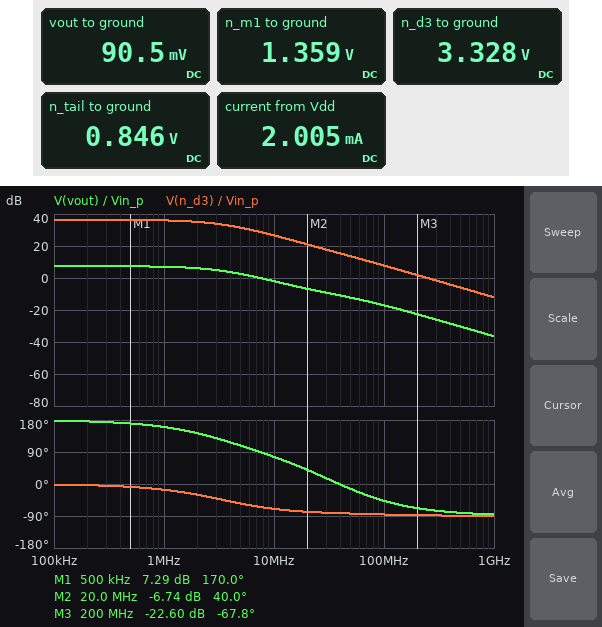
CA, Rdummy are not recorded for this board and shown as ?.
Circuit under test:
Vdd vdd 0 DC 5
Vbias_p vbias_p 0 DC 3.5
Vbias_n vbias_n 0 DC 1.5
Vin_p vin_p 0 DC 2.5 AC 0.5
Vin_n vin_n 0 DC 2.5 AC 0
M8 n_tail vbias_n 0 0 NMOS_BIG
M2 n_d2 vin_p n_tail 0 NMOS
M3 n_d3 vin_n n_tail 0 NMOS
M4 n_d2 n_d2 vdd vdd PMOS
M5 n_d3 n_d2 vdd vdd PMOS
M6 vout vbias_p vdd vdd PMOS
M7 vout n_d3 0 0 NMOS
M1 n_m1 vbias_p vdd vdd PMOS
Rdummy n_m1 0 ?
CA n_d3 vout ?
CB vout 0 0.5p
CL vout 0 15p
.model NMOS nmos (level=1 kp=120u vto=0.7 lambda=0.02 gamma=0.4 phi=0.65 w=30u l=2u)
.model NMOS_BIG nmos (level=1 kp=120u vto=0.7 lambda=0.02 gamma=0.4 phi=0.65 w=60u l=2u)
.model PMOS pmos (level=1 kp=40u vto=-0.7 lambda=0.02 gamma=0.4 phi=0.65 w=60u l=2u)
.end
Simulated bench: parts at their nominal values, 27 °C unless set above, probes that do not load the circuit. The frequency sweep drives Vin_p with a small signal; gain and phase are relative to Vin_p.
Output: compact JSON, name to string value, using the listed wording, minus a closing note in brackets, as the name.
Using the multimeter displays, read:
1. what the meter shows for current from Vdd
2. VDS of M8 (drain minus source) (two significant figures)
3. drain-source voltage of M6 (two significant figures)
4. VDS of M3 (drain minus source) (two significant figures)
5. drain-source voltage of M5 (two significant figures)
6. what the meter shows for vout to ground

{"what the meter shows for current from Vdd": "2.005 mA", "VDS of M8 (drain minus source)": "850 mV", "drain-source voltage of M6": "-4.9 V", "VDS of M3 (drain minus source)": "2.5 V", "drain-source voltage of M5": "-1.7 V", "what the meter shows for vout to ground": "90.5 mV"}
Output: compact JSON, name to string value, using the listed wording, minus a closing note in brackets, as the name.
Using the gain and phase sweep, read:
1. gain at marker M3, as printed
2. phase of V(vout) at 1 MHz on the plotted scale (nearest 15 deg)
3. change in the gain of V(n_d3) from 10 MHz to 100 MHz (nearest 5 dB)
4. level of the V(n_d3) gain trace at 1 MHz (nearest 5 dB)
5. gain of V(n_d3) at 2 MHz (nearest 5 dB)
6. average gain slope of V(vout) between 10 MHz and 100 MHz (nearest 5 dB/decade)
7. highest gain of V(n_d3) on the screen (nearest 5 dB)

{"gain at marker M3, as printed": "-22.60 dB", "phase of V(vout) at 1 MHz on the plotted scale": "165 deg", "change in the gain of V(n_d3) from 10 MHz to 100 MHz": "-20 dB", "level of the V(n_d3) gain trace at 1 MHz": "35 dB", "gain of V(n_d3) at 2 MHz": "35 dB", "average gain slope of V(vout) between 10 MHz and 100 MHz": "-15 dB/decade", "highest gain of V(n_d3) on the screen": "35 dB"}
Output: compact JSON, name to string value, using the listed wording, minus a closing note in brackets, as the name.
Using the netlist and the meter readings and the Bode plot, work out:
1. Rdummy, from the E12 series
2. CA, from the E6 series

{"Rdummy, from the E12 series": "3.3 kΩ", "CA, from the E6 series": "1 pF"}
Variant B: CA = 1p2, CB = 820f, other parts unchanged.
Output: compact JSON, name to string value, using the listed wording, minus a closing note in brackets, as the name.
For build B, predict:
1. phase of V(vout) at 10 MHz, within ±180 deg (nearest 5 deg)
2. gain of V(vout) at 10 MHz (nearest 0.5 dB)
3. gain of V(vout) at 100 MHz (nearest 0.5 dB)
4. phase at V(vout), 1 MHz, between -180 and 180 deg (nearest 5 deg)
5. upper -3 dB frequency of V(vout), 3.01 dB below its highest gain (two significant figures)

{"phase of V(vout) at 10 MHz, within ±180 deg": "70 deg", "gain of V(vout) at 10 MHz": "-3.0 dB", "gain of V(vout) at 100 MHz": "-17.5 dB", "phase at V(vout), 1 MHz, between -180 and 180 deg": "155 deg", "upper -3 dB frequency of V(vout), 3.01 dB below its highest gain": "2.9 MHz"}
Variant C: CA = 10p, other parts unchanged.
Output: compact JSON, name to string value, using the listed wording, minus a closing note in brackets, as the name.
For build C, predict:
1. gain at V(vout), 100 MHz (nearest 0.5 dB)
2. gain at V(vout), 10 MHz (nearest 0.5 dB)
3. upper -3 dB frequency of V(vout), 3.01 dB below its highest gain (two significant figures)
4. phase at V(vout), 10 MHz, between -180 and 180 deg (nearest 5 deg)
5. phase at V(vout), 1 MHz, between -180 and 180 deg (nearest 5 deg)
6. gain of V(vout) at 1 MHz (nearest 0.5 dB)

{"gain at V(vout), 100 MHz": "-17.5 dB", "gain at V(vout), 10 MHz": "-10.0 dB", "upper -3 dB frequency of V(vout), 3.01 dB below its highest gain": "350 kHz", "phase at V(vout), 10 MHz, between -180 and 180 deg": "5 deg", "phase at V(vout), 1 MHz, between -180 and 180 deg": "85 deg", "gain of V(vout) at 1 MHz": "-2.0 dB"}
